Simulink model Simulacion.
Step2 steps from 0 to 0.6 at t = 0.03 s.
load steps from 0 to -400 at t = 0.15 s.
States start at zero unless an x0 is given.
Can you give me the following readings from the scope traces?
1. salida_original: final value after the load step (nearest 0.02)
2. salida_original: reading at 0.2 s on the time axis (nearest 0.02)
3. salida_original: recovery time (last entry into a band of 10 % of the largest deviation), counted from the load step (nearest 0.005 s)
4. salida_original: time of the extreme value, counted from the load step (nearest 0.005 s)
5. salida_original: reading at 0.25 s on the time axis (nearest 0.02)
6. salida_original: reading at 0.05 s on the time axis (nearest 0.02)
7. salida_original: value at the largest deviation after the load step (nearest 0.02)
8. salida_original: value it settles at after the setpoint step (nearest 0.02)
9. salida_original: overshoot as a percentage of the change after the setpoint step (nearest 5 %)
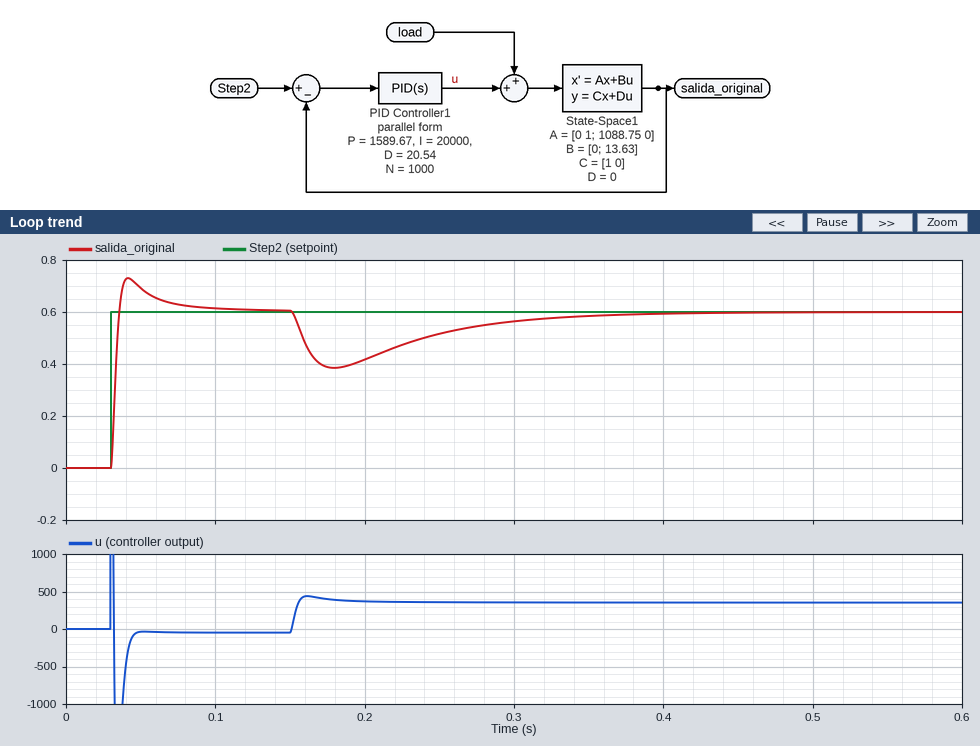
0.60
0.42
0.180 s
0.030 s
0.52
0.70
0.38
0.60
20 %
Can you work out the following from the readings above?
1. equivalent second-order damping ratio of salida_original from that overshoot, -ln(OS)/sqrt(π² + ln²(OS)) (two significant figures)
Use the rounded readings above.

0.46
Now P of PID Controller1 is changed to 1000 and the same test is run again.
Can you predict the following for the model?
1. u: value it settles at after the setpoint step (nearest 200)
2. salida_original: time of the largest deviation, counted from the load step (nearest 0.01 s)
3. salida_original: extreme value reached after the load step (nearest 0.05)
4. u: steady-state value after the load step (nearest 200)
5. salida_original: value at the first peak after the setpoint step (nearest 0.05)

0
0.04 s
0.30
400
0.70
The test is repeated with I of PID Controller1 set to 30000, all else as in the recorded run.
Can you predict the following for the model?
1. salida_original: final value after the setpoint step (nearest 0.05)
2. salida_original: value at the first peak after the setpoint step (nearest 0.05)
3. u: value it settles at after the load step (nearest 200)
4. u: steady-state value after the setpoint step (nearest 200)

0.60
0.75
400
0
